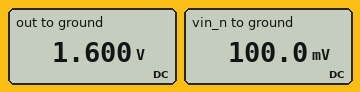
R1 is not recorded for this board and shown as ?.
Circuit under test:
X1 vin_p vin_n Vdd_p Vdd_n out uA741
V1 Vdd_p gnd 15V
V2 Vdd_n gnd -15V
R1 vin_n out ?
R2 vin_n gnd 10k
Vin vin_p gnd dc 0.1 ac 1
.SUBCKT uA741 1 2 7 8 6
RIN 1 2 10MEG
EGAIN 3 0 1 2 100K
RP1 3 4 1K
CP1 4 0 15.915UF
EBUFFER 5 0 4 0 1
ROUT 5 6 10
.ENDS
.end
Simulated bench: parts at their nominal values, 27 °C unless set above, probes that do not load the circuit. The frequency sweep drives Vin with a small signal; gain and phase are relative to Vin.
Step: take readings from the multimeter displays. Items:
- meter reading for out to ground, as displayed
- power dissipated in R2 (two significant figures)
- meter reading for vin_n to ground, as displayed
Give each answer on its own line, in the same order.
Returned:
1.600 V
1.0 µW
100.0 mV
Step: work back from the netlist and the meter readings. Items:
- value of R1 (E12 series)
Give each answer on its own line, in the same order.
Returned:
150 kΩ
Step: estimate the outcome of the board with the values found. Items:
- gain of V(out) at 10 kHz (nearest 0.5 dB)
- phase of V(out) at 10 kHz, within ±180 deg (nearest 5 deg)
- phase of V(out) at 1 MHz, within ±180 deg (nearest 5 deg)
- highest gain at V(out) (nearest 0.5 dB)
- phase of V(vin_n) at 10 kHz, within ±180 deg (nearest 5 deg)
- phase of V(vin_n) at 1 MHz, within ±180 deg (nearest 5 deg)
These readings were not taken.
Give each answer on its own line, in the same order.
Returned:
24.0 dB
-10 deg
-85 deg
24.0 dB
-10 deg
-85 deg
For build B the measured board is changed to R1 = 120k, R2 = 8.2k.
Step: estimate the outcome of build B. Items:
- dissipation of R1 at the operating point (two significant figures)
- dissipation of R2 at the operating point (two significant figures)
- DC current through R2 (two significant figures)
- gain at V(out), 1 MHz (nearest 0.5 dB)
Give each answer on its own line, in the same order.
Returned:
18 µW
1.2 µW
12 µA
0 dB
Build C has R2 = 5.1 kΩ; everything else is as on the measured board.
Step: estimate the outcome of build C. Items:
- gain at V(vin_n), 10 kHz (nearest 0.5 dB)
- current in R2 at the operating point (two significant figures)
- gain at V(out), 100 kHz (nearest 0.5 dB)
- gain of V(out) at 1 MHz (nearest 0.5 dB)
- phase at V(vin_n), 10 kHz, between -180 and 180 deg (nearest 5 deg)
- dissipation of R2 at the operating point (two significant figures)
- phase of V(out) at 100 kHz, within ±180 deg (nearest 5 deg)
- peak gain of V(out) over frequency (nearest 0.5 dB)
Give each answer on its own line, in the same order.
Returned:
-0.5 dB
20 µA
19.5 dB
0 dB
-15 deg
2.0 µW
-70 deg
29.5 dB
